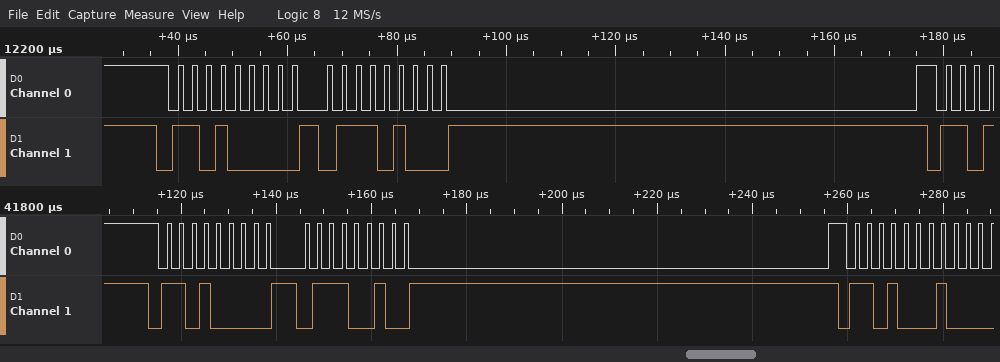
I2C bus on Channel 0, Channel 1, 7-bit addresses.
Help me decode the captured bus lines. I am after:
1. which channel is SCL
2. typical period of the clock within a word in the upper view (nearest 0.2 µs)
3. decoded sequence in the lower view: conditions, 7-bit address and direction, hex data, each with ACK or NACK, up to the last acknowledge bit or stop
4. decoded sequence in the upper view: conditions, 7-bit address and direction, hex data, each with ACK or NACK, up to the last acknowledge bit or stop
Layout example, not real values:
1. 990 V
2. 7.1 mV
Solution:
1. Channel 0
2. 2.6 µs
3. start, address 68 write ACK, 72 ACK, repeated start, address 68 read ACK
4. start, address 68 write ACK, 74 ACK
